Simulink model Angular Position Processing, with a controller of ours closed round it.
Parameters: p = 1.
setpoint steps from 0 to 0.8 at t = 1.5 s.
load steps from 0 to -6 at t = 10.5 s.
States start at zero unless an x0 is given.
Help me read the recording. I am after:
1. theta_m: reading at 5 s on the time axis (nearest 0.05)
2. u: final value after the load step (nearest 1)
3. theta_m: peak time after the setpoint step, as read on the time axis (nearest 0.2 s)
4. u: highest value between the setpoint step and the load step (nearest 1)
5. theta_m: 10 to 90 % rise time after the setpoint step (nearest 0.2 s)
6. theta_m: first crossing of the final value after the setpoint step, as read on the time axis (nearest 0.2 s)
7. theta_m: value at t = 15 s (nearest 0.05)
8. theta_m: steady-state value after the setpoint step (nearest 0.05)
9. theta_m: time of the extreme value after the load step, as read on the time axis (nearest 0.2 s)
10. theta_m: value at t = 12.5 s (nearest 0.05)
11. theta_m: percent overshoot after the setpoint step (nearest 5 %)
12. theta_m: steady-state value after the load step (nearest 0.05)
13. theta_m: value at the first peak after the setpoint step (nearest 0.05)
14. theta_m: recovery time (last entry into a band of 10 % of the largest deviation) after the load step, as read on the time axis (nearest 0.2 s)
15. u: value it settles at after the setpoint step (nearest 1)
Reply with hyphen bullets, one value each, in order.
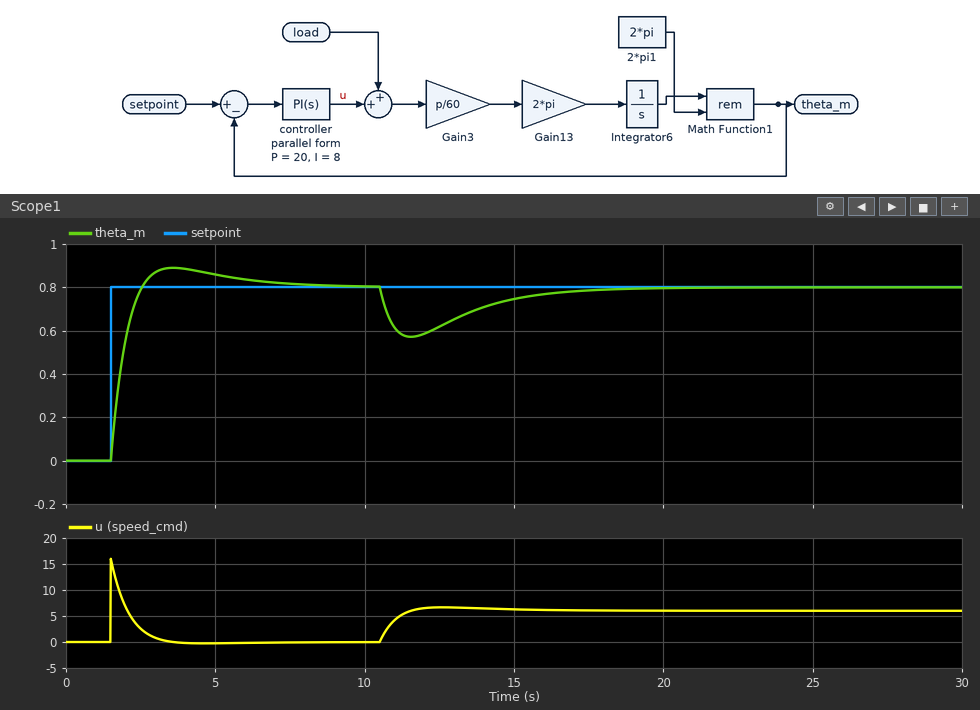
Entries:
- 0.85
- 6
- 3.6 s
- 16
- 0.8 s
- 2.6 s
- 0.75
- 0.80
- 11.6 s
- 0.60
- 10 %
- 0.80
- 0.90
- 16.6 s
- 0
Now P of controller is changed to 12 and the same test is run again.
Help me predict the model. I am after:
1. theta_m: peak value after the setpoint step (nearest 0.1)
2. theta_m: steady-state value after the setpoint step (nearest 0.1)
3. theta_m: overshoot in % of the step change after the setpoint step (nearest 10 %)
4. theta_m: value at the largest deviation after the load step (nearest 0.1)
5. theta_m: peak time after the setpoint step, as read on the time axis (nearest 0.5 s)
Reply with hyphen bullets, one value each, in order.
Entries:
- 1.0
- 0.8
- 20 %
- 0.5
- 4.0 s
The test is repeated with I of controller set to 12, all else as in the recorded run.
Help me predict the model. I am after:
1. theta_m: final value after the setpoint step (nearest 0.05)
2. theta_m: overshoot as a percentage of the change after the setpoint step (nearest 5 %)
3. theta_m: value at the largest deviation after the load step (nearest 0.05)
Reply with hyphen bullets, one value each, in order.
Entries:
- 0.80
- 15 %
- 0.60
